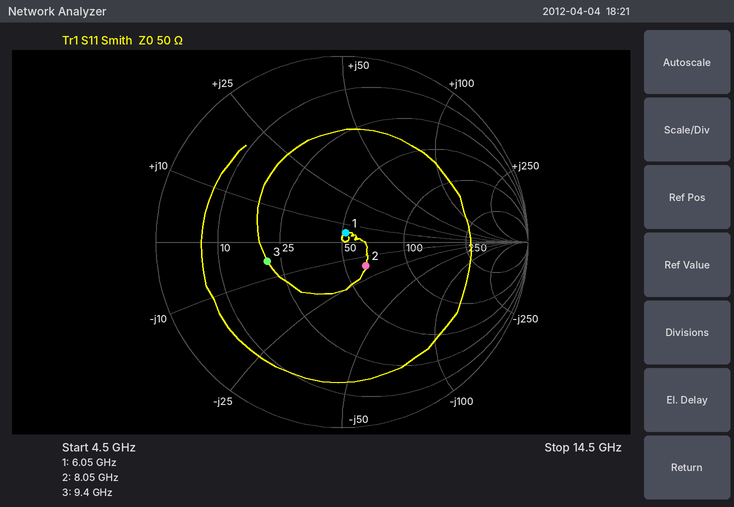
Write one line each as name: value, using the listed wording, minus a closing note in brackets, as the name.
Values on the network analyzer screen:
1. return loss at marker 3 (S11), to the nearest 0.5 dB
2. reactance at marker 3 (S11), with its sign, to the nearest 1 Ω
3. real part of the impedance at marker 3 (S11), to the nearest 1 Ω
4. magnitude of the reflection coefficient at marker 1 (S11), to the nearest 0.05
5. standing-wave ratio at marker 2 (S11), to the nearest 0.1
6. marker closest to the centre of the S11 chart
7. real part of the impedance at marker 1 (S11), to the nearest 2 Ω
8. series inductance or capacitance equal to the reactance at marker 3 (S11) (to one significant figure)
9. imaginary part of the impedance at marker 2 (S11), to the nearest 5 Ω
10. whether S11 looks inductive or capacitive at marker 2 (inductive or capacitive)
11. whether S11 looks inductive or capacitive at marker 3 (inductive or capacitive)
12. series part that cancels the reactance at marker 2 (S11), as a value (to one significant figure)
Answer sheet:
return loss at marker 3 (S11), to the nearest 0.5 dB: 7.5 dB
reactance at marker 3 (S11), with its sign, to the nearest 1 Ω: -5 Ω
real part of the impedance at marker 3 (S11), to the nearest 1 Ω: 21 Ω
magnitude of the reflection coefficient at marker 1 (S11), to the nearest 0.05: 0.05
standing-wave ratio at marker 2 (S11), to the nearest 0.1: 1.4
marker closest to the centre of the S11 chart: marker 1
real part of the impedance at marker 1 (S11), to the nearest 2 Ω: 52 Ω
series inductance or capacitance equal to the reactance at marker 3 (S11): 3 pF
imaginary part of the impedance at marker 2 (S11), to the nearest 5 Ω: -15 Ω
whether S11 looks inductive or capacitive at marker 2: capacitive
whether S11 looks inductive or capacitive at marker 3: capacitive
series part that cancels the reactance at marker 2 (S11), as a value: 300 pH
